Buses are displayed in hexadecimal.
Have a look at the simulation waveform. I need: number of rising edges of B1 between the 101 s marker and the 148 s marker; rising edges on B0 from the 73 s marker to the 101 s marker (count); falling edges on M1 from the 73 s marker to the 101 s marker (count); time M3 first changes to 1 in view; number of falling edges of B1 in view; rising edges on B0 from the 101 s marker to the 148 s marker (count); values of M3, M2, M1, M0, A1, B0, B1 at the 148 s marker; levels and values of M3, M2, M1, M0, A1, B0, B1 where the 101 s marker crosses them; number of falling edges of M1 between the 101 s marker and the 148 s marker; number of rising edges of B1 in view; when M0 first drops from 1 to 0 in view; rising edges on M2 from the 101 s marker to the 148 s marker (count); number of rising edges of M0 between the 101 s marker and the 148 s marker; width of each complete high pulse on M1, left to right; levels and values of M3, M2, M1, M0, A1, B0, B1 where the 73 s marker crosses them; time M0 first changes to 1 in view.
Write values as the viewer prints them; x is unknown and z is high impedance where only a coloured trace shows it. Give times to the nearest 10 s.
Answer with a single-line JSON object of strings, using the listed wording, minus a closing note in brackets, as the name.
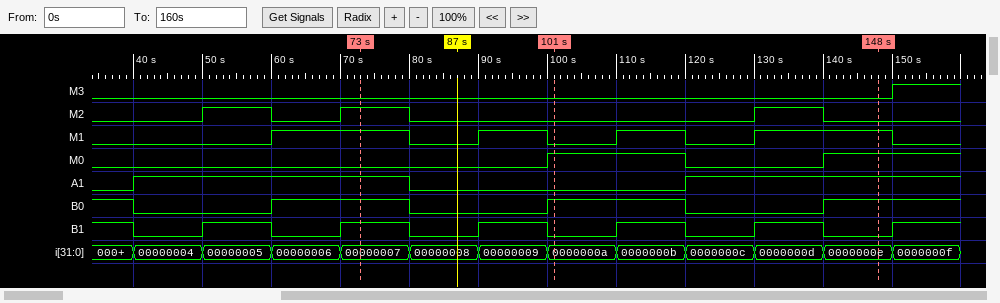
{"number of rising edges of B1 between the 101 s marker and the 148 s marker": "2", "rising edges on B0 from the 73 s marker to the 101 s marker": "1", "falling edges on M1 from the 73 s marker to the 101 s marker": "2", "time M3 first changes to 1 in view": "150 s", "number of falling edges of B1 in view": "6", "rising edges on B0 from the 101 s marker to the 148 s marker": "1", "values of M3, M2, M1, M0, A1, B0, B1 at the 148 s marker": "M3=0, M2=0, M1=1, M0=1, A1=1, B0=1, B1=0", "levels and values of M3, M2, M1, M0, A1, B0, B1 where the 101 s marker crosses them": "M3=0, M2=0, M1=0, M0=1, A1=0, B0=1, B1=0", "number of falling edges of M1 between the 101 s marker and the 148 s marker": "1", "number of rising edges of B1 in view": "6", "when M0 first drops from 1 to 0 in view": "120 s", "rising edges on M2 from the 101 s marker to the 148 s marker": "1", "number of rising edges of M0 between the 101 s marker and the 148 s marker": "1", "width of each complete high pulse on M1, left to right": "20 s, 10 s, 10 s, 20 s", "levels and values of M3, M2, M1, M0, A1, B0, B1 where the 73 s marker crosses them": "M3=0, M2=1, M1=1, M0=0, A1=1, B0=1, B1=1", "time M0 first changes to 1 in view": "100 s"}
